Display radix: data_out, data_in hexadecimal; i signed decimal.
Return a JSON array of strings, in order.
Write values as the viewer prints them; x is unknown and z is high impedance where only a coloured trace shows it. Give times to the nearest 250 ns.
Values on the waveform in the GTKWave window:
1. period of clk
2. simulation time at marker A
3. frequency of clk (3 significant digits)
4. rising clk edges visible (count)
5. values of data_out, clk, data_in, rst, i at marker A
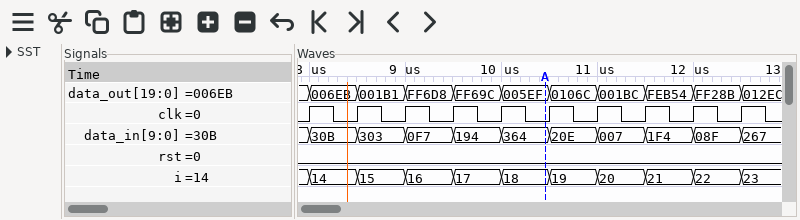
["500 ns", "10500 ns", "2.00 MHz", "10", "data_out=005EF, clk=0, data_in=364, rst=0, i=18"]
